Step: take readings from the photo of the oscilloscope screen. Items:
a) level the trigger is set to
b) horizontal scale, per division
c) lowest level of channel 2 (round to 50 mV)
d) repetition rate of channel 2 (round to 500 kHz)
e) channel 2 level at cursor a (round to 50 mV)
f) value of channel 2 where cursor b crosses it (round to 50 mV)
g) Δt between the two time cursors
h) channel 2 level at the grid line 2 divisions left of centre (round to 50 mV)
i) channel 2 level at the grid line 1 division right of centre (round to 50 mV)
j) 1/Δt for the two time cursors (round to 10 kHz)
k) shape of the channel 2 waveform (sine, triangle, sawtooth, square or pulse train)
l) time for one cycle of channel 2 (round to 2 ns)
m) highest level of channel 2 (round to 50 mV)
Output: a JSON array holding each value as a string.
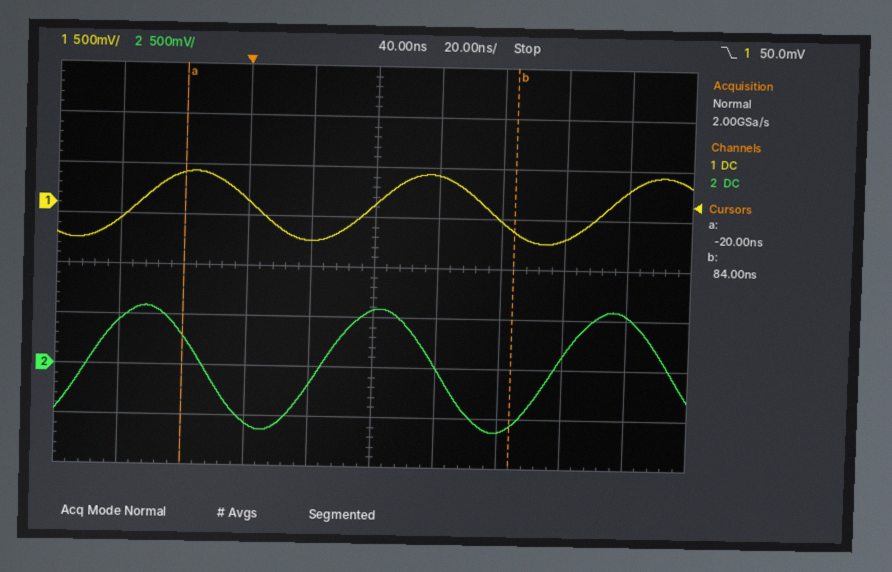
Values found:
["50.0 mV", "20 ns", "-650 mV", "13.5 MHz", "300 mV", "-550 mV", "104 ns", "-550 mV", "0 mV", "9.62 MHz", "sine", "74 ns", "600 mV"]
